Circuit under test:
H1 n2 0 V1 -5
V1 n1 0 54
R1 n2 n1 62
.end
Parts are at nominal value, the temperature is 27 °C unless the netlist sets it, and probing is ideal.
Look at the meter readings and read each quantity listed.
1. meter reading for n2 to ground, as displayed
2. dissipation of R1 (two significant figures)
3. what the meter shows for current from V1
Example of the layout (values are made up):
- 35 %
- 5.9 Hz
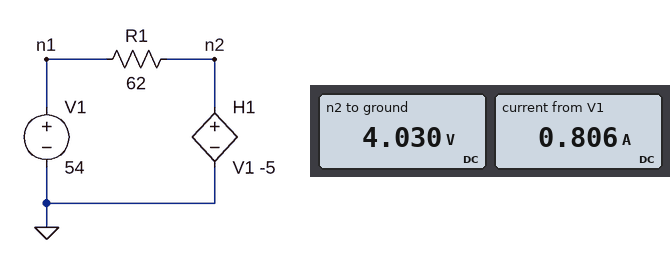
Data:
- 4.030 V
- 40 W
- 0.806 A
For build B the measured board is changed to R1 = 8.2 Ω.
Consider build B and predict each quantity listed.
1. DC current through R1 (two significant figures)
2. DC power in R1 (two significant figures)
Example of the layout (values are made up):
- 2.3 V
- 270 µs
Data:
- 4.1 A
- 140 W
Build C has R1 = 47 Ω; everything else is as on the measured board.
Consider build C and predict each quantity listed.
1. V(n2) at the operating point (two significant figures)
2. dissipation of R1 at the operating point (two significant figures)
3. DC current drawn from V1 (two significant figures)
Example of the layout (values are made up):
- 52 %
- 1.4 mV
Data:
- 5.2 V
- 51 W
- 1.0 A
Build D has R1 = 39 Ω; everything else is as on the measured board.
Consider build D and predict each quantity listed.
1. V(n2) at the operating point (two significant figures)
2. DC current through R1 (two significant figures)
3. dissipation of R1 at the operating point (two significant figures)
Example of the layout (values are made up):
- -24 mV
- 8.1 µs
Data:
- 6.1 V
- 1.2 A
- 59 W
